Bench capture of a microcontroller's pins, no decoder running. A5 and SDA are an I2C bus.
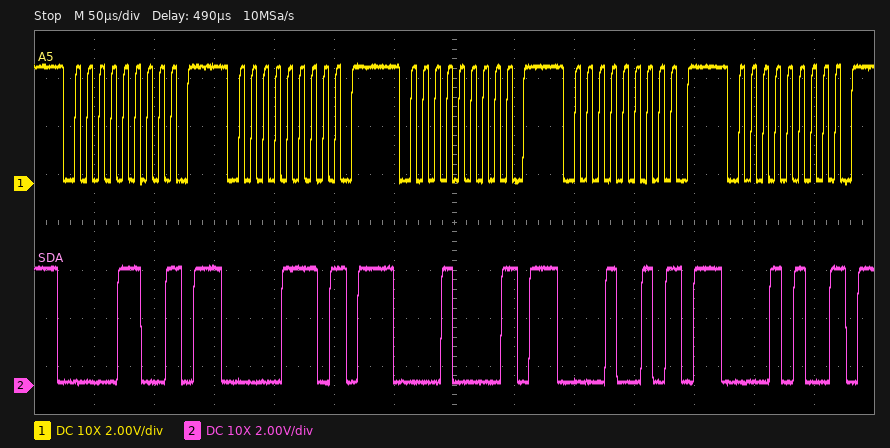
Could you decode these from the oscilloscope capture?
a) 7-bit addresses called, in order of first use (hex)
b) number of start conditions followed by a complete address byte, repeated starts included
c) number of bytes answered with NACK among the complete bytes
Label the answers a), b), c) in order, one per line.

a) 0x06 0x07 0x08 0x09 0x0A
b) 5
c) 5
